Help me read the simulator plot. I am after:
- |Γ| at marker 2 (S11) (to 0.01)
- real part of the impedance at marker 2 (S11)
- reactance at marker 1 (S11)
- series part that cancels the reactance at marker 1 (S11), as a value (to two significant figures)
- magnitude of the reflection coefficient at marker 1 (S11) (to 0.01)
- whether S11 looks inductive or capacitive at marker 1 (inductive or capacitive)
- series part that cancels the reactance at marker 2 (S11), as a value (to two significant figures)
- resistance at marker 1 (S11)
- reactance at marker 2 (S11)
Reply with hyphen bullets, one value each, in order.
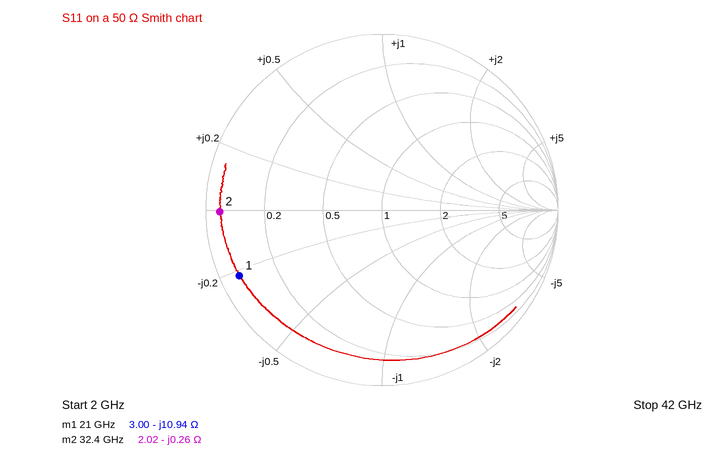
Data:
- 0.92
- 2.02 Ω
- -10.94 Ω
- 83 pH
- 0.89
- capacitive
- 1.3 pH
- 3.00 Ω
- -0.26 Ω
